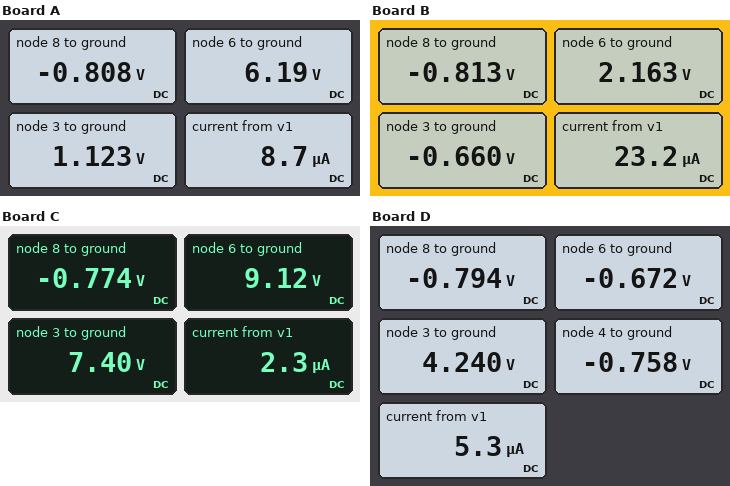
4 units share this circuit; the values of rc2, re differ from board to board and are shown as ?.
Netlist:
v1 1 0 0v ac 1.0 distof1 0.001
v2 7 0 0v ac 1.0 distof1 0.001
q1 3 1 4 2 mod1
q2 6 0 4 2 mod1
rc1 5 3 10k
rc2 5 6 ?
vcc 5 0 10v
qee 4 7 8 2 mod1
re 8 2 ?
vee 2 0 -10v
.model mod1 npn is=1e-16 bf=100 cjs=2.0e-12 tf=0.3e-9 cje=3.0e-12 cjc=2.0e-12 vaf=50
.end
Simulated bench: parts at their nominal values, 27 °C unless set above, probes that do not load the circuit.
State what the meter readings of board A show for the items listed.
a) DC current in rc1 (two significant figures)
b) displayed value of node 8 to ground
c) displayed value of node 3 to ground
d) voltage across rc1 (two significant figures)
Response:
890 µA
-0.808 V
1.123 V
8.9 V
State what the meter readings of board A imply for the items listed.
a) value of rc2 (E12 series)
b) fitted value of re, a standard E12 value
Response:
3.9 kΩ
3.3 kΩ
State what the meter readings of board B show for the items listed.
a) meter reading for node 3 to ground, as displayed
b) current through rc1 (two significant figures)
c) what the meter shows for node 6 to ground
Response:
-0.660 V
1.1 mA
2.163 V
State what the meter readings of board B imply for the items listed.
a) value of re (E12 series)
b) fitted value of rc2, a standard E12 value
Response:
2.7 kΩ
6.8 kΩ
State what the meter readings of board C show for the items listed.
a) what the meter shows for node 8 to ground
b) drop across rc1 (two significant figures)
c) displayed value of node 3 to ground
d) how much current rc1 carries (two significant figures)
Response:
-0.774 V
2.6 V
7.40 V
260 µA
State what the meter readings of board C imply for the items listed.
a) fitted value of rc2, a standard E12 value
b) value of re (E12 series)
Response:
3.3 kΩ
12 kΩ
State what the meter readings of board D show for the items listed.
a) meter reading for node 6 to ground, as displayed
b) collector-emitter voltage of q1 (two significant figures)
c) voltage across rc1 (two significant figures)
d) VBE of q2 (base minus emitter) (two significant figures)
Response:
-0.672 V
5.0 V
5.8 V
760 mV
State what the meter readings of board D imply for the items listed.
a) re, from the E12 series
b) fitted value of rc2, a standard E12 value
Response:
5.6 kΩ
22 kΩ
